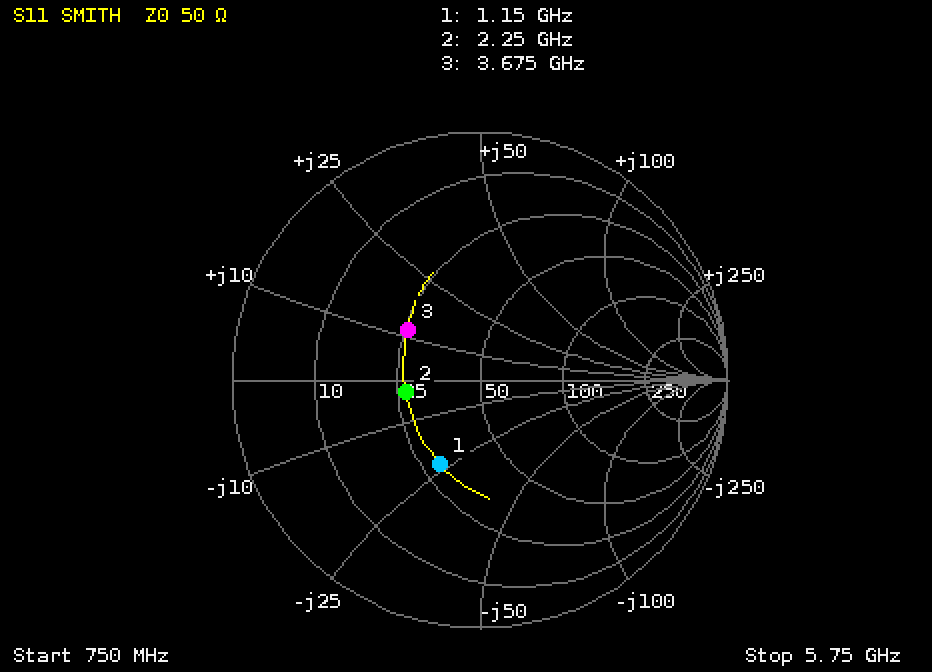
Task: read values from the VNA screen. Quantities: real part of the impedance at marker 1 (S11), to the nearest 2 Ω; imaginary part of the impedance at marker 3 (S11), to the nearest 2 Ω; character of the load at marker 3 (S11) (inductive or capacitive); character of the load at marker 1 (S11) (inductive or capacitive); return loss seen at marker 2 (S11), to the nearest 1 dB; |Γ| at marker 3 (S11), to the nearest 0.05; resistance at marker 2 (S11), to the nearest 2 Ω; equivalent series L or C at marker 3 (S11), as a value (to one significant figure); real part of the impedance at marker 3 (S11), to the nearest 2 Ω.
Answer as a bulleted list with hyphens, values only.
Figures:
- 30 Ω
- +12 Ω
- inductive
- capacitive
- 10 dB
- 0.35
- 26 Ω
- 500 pH
- 26 Ω
